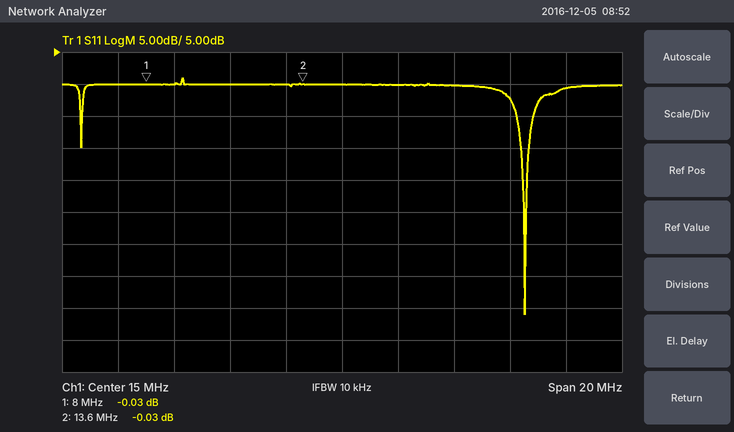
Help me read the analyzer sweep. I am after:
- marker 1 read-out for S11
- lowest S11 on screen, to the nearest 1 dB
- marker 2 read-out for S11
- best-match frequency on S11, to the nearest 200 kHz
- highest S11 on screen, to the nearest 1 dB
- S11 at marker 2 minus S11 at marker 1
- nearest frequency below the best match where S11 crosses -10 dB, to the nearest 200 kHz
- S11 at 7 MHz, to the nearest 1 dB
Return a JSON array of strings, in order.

["-0.03 dB", "-36 dB", "-0.03 dB", "21.6 MHz", "1 dB", "0.00 dB", "21.4 MHz", "0 dB"]
